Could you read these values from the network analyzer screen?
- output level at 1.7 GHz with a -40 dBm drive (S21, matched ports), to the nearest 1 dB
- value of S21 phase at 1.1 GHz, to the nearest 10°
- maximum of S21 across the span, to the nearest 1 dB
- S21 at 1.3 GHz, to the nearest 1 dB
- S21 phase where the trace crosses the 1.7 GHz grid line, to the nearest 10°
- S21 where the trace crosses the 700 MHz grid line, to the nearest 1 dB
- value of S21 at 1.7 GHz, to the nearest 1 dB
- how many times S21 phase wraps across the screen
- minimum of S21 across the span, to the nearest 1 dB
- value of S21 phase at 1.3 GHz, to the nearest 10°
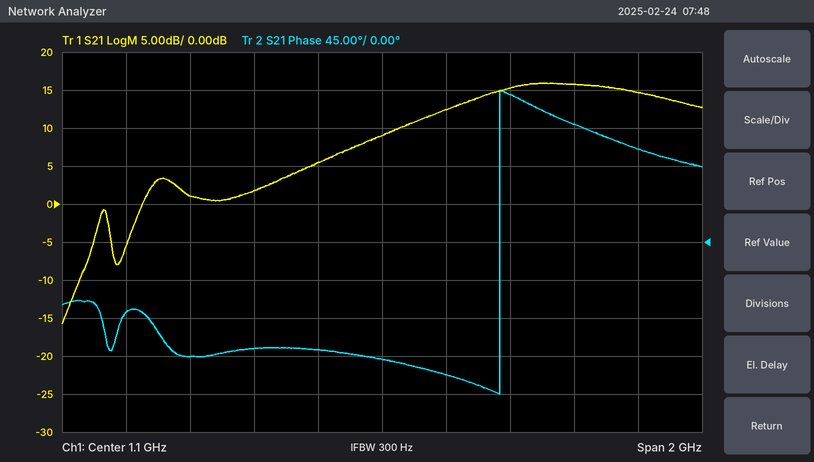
-24 dBm
-140°
16 dB
12 dB
140°
2 dB
16 dB
1
-16 dB
-160°
